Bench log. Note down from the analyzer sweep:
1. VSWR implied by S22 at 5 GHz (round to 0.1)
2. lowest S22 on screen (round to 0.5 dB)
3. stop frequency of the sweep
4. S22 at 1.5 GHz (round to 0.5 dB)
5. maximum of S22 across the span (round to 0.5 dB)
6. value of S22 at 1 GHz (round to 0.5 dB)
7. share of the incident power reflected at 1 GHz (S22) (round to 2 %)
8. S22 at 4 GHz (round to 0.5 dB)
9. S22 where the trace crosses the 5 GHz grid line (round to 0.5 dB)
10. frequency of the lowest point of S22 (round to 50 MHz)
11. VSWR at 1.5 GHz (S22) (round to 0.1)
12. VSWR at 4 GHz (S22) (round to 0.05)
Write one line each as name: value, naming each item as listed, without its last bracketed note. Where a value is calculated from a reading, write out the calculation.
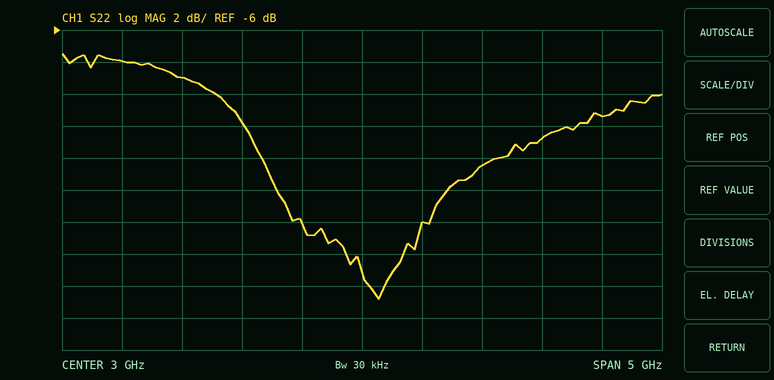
VSWR implied by S22 at 5 GHz: |Γ| = 10^(-11.5/20) = 0.2661; VSWR = (1 + 0.2661)/(1 − 0.2661) ≈ 1.7
lowest S22 on screen: -23.0 dB
stop frequency of the sweep: 5.5 GHz
S22 at 1.5 GHz: -9.0 dB
maximum of S22 across the span: -7.5 dB
value of S22 at 1 GHz: -8.0 dB
share of the incident power reflected at 1 GHz (S22): 10^(-8/10) ≈ 16 %
S22 at 4 GHz: -14.5 dB
S22 where the trace crosses the 5 GHz grid line: -11.5 dB
frequency of the lowest point of S22: 3.15 GHz
VSWR at 1.5 GHz (S22): |Γ| = 10^(-9/20) = 0.3548; VSWR = (1 + 0.3548)/(1 − 0.3548) ≈ 2.1
VSWR at 4 GHz (S22): |Γ| = 10^(-14.5/20) = 0.1884; VSWR = (1 + 0.1884)/(1 − 0.1884) ≈ 1.46, so 1.45 to the nearest 0.05
